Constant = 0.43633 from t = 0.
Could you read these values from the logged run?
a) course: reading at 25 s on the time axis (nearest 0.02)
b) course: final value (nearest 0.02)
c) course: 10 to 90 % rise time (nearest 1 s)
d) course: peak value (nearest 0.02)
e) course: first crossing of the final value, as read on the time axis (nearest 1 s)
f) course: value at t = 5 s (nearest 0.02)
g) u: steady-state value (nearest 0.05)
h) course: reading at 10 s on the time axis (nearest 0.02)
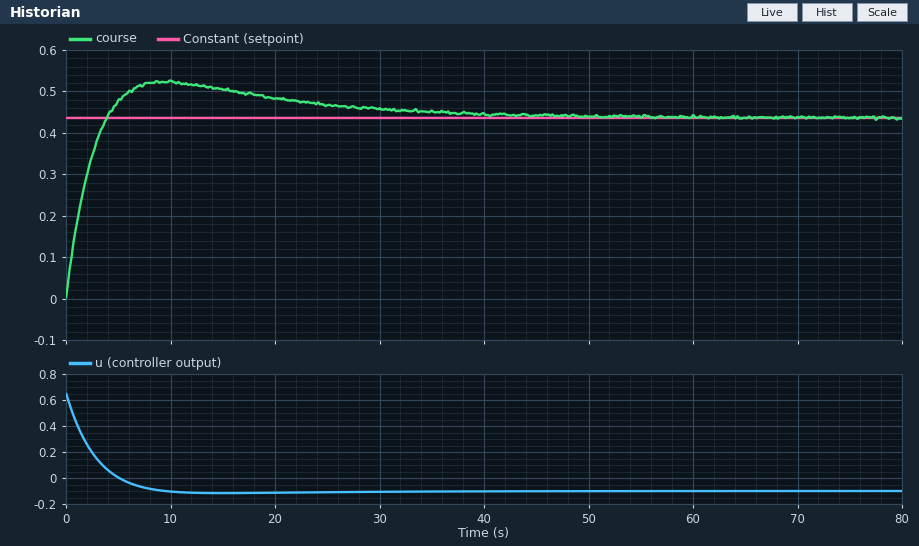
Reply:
0.46
0.44
3 s
0.52
4 s
0.48
-0.10
0.52
